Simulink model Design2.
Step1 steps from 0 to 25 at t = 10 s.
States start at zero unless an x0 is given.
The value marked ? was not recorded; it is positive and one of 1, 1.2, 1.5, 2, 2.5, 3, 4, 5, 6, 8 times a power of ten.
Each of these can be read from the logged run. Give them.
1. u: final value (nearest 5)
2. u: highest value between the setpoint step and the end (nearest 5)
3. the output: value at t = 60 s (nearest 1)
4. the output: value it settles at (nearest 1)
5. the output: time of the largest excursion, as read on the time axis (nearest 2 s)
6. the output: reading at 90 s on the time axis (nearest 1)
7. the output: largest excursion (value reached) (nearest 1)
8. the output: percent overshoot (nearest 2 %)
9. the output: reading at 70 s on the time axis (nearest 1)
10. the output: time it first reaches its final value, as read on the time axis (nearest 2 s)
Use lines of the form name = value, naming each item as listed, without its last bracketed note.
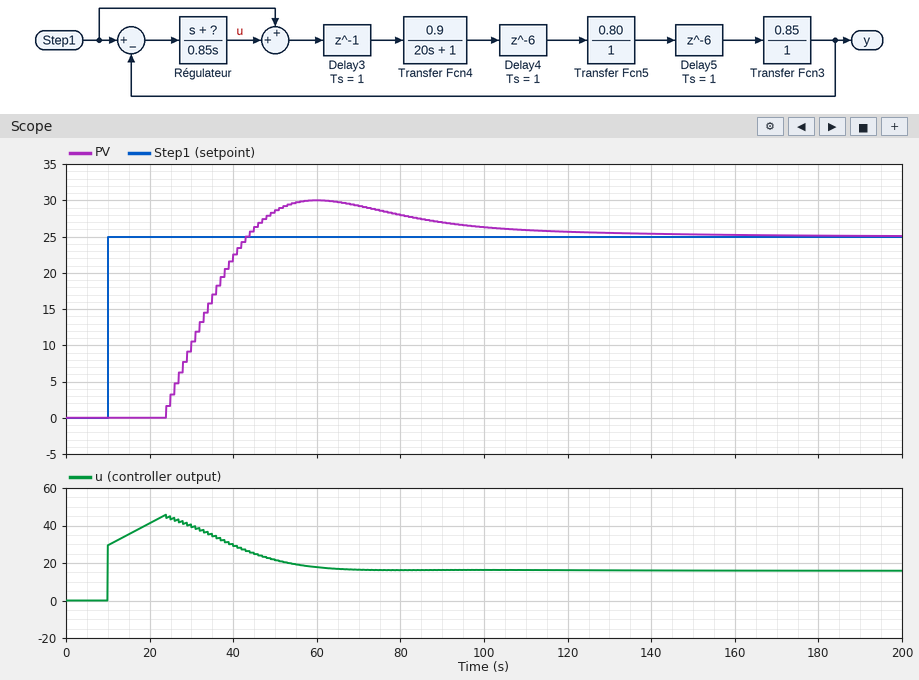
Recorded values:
u: final value = 15
u: highest value between the setpoint step and the end = 45
the output: value at t = 60 s = 30
the output: value it settles at = 25
the output: time of the largest excursion, as read on the time axis = 60 s
the output: reading at 90 s on the time axis = 27
the output: largest excursion (value reached) = 30
the output: percent overshoot = 20 %
the output: reading at 70 s on the time axis = 29
the output: time it first reaches its final value, as read on the time axis = 44 s
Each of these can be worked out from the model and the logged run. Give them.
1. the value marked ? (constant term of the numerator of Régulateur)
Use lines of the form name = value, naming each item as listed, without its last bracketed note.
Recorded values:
the value marked ? = 0.04
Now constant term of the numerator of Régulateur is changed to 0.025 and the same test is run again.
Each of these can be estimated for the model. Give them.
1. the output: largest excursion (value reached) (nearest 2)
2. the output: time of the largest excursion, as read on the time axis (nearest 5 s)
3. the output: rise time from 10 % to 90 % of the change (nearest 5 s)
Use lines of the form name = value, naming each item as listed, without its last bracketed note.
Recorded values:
the output: largest excursion (value reached) = 26
the output: time of the largest excursion, as read on the time axis = 60 s
the output: rise time from 10 % to 90 % of the change = 15 s
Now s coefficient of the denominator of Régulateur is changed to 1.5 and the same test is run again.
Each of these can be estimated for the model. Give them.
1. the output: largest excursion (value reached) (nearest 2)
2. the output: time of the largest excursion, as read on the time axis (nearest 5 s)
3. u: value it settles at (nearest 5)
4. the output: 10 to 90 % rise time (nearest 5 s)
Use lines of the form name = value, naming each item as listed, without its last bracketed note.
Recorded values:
the output: largest excursion (value reached) = 26
the output: time of the largest excursion, as read on the time axis = 90 s
u: value it settles at = 15
the output: 10 to 90 % rise time = 25 s
